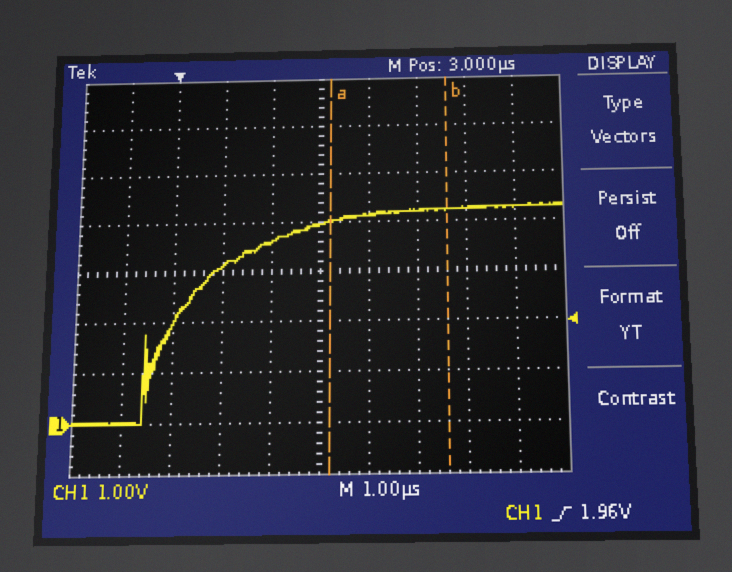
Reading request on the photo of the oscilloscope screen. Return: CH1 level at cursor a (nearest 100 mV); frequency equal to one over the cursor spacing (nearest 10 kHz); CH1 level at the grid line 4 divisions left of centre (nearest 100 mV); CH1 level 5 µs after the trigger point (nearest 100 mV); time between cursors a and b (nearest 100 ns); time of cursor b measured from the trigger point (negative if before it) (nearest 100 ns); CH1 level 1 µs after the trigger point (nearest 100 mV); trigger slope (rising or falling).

4.0 V
420 kHz
0.0 V
4.2 V
2.4 µs
+5.6 µs
3.1 V
rising
